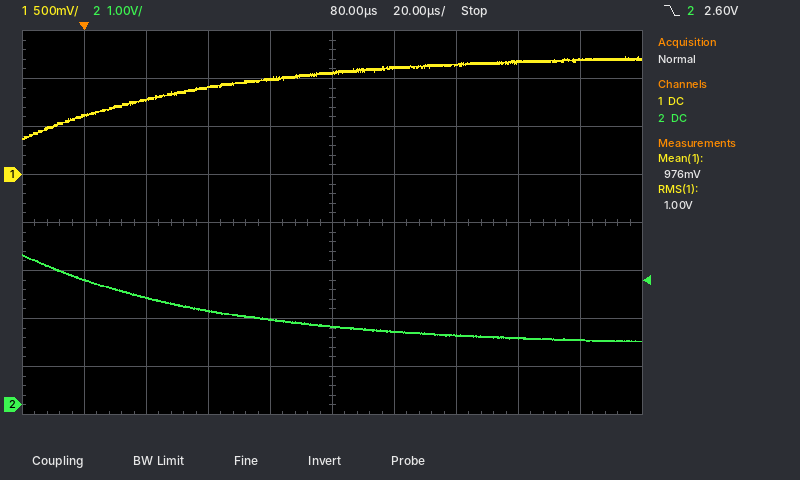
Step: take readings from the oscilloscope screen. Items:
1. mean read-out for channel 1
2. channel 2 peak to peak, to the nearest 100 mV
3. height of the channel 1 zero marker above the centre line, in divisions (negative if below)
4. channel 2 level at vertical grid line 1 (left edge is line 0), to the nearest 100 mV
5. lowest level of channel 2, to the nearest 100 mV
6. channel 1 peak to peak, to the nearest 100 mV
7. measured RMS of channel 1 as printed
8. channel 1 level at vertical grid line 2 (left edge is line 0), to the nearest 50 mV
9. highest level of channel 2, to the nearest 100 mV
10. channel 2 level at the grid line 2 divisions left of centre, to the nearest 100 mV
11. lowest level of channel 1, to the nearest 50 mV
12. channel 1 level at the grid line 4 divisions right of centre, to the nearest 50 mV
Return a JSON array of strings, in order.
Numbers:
["976 mV", "1.8 V", "+1.0 div", "2.6 V", "1.3 V", "900 mV", "1.00 V", "800 mV", "3.1 V", "2.0 V", "350 mV", "1.20 V"]
